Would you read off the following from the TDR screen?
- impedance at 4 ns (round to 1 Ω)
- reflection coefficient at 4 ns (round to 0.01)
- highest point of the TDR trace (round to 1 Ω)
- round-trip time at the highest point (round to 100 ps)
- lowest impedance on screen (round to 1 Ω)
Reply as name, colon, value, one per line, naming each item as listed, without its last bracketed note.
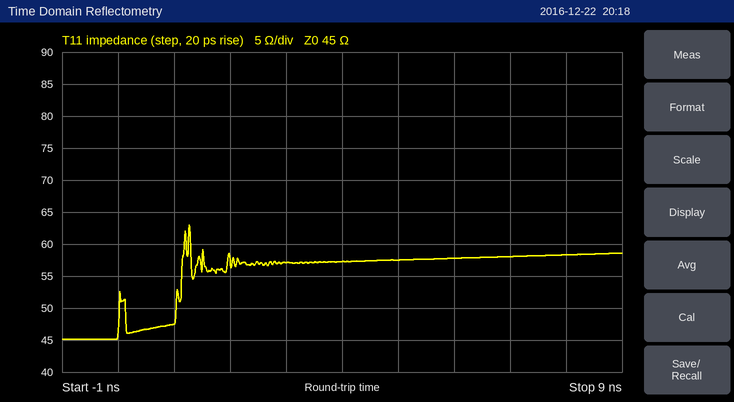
impedance at 4 ns: 57 Ω
reflection coefficient at 4 ns: +0.12
highest point of the TDR trace: 63 Ω
round-trip time at the highest point: 1.3 ns
lowest impedance on screen: 45 Ω
